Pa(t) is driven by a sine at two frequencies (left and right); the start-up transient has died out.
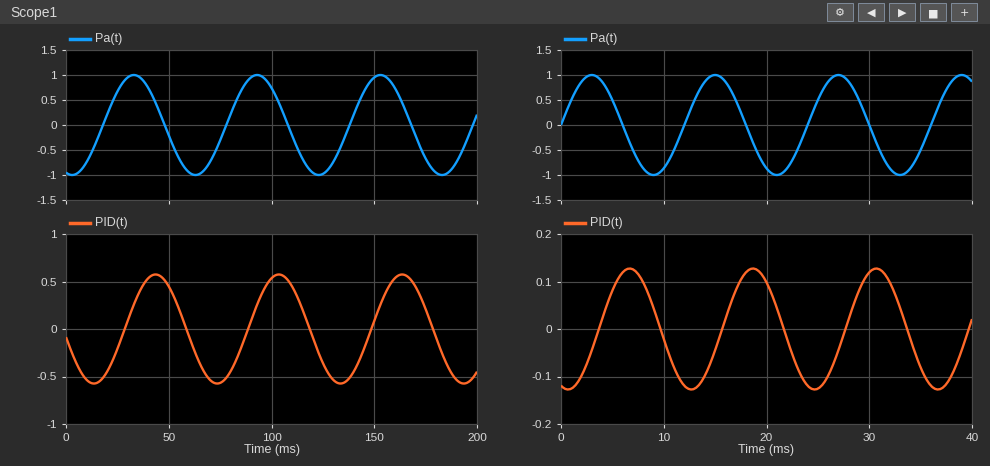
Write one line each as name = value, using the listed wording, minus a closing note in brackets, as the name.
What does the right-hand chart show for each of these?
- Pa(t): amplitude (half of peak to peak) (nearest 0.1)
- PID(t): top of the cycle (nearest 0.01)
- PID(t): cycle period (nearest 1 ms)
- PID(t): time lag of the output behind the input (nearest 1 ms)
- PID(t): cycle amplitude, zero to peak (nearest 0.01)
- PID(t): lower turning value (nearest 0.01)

Pa(t): amplitude (half of peak to peak) = 1.0
PID(t): top of the cycle = 0.13
PID(t): cycle period = 12 ms
PID(t): time lag of the output behind the input = 4 ms
PID(t): cycle amplitude, zero to peak = 0.13
PID(t): lower turning value = -0.13
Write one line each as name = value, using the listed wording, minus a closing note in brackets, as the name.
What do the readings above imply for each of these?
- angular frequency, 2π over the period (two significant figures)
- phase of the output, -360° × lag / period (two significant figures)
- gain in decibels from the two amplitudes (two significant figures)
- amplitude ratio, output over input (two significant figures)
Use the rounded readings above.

angular frequency, 2π over the period = 0.52 rad/ms
phase of the output, -360° × lag / period = -120°
gain in decibels from the two amplitudes = -18 dB
amplitude ratio, output over input = 0.13
